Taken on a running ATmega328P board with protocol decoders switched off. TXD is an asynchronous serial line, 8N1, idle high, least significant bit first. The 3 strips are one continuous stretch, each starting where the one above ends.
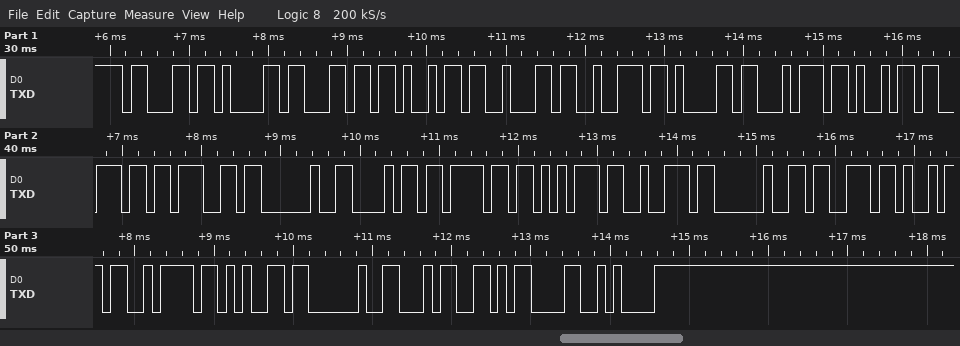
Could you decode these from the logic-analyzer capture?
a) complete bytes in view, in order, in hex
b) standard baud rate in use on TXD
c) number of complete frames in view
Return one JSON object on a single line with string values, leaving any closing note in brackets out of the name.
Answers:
{"complete bytes in view, in order, in hex": "63 61 6C 69 62 72 61 74 69 6E 67 20 68 6F 75 72 20 73 69 7A 65 20 34 0D 0A", "standard baud rate in use on TXD": "9600 baud", "number of complete frames in view": "25"}
